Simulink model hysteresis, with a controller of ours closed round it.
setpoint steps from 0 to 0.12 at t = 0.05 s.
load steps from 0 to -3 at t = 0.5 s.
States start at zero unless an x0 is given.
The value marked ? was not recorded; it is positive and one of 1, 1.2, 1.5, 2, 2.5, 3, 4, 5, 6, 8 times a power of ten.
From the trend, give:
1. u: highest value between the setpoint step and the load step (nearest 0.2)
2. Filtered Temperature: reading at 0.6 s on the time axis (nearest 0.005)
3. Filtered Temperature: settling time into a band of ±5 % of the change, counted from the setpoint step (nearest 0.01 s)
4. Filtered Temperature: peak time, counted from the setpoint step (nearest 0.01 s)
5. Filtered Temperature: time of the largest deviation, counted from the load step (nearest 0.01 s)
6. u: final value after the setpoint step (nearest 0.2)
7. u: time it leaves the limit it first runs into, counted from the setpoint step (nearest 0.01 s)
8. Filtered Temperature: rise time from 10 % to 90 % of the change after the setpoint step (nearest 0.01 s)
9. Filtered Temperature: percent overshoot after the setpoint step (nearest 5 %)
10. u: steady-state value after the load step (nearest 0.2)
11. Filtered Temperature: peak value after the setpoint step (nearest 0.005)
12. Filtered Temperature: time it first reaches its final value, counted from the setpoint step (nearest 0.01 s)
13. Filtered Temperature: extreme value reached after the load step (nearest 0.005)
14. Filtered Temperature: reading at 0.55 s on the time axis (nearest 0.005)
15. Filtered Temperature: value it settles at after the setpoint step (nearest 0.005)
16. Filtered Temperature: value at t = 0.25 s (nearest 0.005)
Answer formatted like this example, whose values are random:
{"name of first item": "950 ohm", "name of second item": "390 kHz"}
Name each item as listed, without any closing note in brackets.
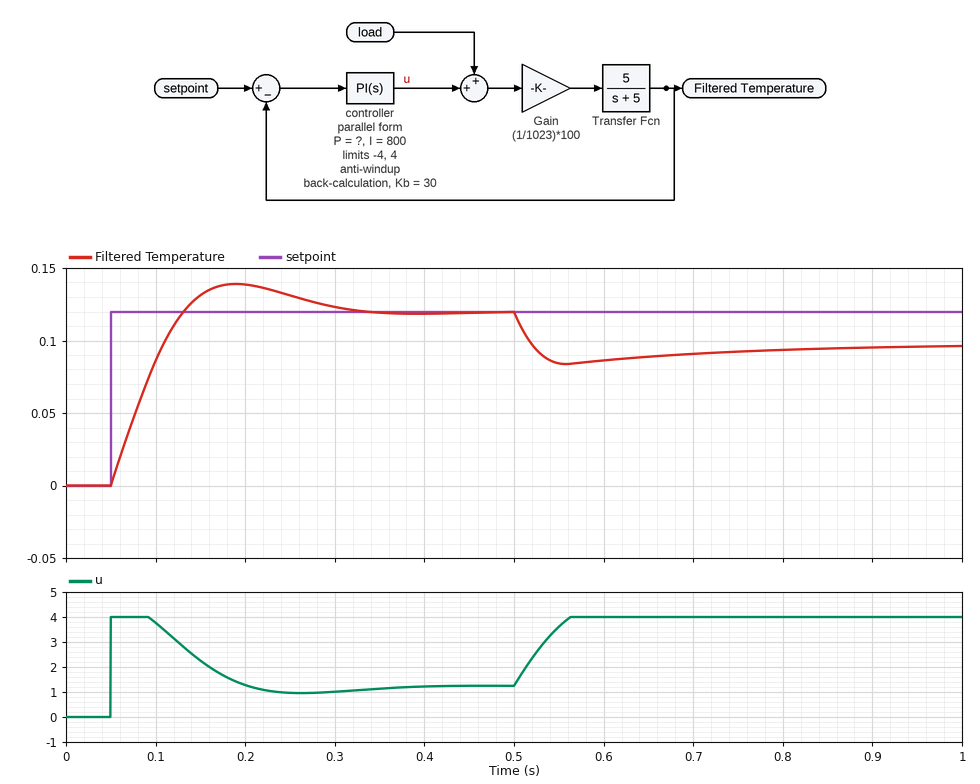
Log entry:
{"u: highest value between the setpoint step and the load step": "4.0", "Filtered Temperature: reading at 0.6 s on the time axis": "0.085", "Filtered Temperature: settling time into a band of ±5 % of the change, counted from the setpoint step": "0.23 s", "Filtered Temperature: peak time, counted from the setpoint step": "0.14 s", "Filtered Temperature: time of the largest deviation, counted from the load step": "0.06 s", "u: final value after the setpoint step": "1.2", "u: time it leaves the limit it first runs into, counted from the setpoint step": "0.04 s", "Filtered Temperature: rise time from 10 % to 90 % of the change after the setpoint step": "0.06 s", "Filtered Temperature: percent overshoot after the setpoint step": "15 %", "u: steady-state value after the load step": "4.0", "Filtered Temperature: peak value after the setpoint step": "0.140", "Filtered Temperature: time it first reaches its final value, counted from the setpoint step": "0.08 s", "Filtered Temperature: extreme value reached after the load step": "0.085", "Filtered Temperature: reading at 0.55 s on the time axis": "0.085", "Filtered Temperature: value it settles at after the setpoint step": "0.120", "Filtered Temperature: value at t = 0.25 s": "0.130"}
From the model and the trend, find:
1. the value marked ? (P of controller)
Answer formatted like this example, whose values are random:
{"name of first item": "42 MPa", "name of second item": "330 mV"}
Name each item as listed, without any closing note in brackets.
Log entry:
{"the value marked ?": "40"}
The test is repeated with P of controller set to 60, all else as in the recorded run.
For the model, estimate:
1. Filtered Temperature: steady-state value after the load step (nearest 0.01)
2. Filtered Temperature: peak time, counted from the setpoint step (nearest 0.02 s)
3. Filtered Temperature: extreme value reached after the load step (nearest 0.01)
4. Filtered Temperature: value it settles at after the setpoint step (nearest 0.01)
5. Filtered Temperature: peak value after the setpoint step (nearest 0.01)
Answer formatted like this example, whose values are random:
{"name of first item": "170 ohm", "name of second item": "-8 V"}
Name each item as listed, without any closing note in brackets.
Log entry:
{"Filtered Temperature: steady-state value after the load step": "0.10", "Filtered Temperature: peak time, counted from the setpoint step": "0.16 s", "Filtered Temperature: extreme value reached after the load step": "0.09", "Filtered Temperature: value it settles at after the setpoint step": "0.12", "Filtered Temperature: peak value after the setpoint step": "0.13"}
